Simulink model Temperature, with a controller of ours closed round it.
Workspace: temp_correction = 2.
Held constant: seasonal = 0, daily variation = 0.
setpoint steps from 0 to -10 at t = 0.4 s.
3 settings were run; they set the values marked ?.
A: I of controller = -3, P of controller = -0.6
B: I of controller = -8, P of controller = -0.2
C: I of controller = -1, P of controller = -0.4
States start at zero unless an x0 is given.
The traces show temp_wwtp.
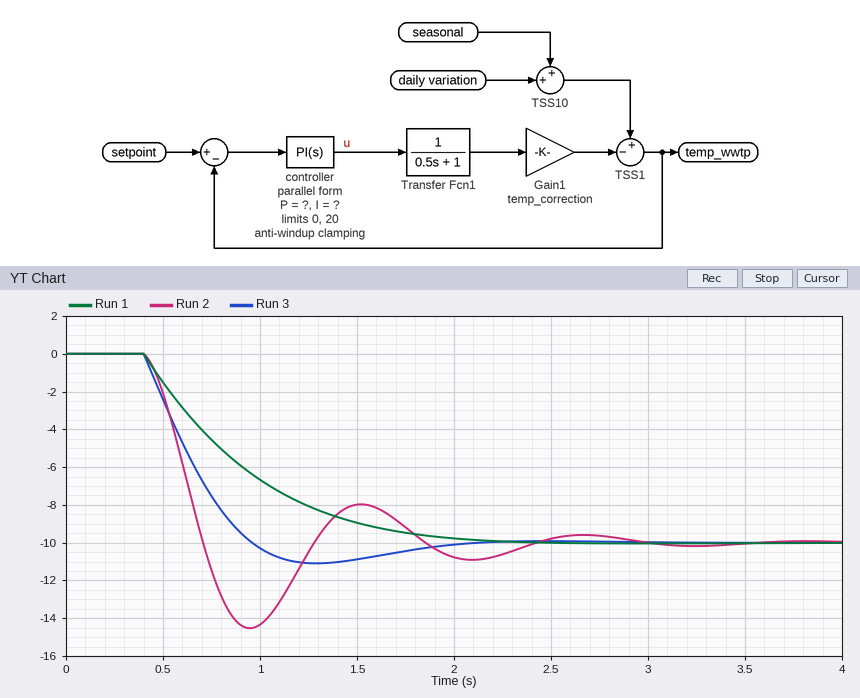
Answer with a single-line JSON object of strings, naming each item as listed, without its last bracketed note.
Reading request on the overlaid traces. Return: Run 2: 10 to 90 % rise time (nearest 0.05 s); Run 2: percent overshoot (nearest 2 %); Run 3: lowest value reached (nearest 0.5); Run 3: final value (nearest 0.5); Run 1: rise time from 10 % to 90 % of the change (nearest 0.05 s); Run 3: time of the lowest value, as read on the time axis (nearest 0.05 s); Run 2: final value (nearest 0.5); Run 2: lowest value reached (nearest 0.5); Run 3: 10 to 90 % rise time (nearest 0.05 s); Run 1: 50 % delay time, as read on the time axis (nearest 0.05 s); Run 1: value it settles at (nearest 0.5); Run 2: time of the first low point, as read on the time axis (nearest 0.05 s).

{"Run 2: 10 to 90 % rise time": "0.20 s", "Run 2: percent overshoot": "46 %", "Run 3: lowest value reached": "-11.0", "Run 3: final value": "-10.0", "Run 1: rise time from 10 % to 90 % of the change": "1.05 s", "Run 3: time of the lowest value, as read on the time axis": "1.30 s", "Run 2: final value": "-10.0", "Run 2: lowest value reached": "-14.5", "Run 3: 10 to 90 % rise time": "0.40 s", "Run 1: 50 % delay time, as read on the time axis": "0.80 s", "Run 1: value it settles at": "-10.0", "Run 2: time of the first low point, as read on the time axis": "0.95 s"}
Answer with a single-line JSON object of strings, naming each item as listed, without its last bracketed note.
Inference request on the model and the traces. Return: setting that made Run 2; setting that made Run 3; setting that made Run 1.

{"setting that made Run 2": "B", "setting that made Run 3": "A", "setting that made Run 1": "C"}
